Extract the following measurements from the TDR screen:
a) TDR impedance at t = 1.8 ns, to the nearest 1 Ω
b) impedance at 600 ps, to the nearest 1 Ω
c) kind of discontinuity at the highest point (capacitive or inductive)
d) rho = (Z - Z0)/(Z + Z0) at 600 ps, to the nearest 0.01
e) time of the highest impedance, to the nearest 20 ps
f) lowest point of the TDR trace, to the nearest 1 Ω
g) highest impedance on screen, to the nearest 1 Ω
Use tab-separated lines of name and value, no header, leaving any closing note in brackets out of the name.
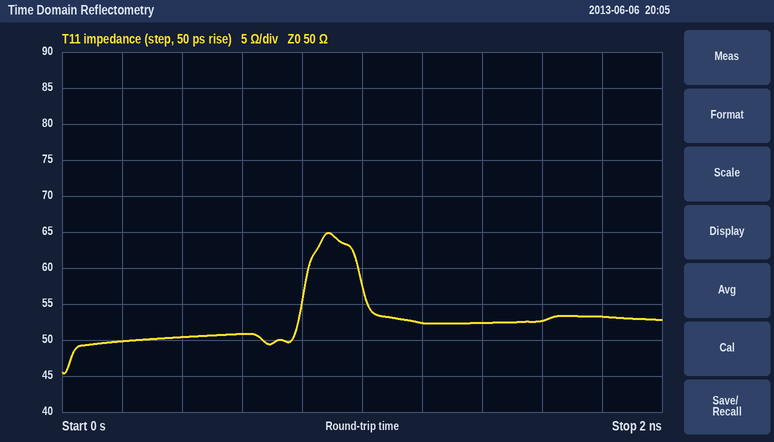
TDR impedance at t = 1.8 ns, to the nearest 1 Ω	53 Ω
impedance at 600 ps, to the nearest 1 Ω	51 Ω
kind of discontinuity at the highest point	inductive
rho = (Z - Z0)/(Z + Z0) at 600 ps, to the nearest 0.01	+0.01
time of the highest impedance, to the nearest 20 ps	880 ps
lowest point of the TDR trace, to the nearest 1 Ω	45 Ω
highest impedance on screen, to the nearest 1 Ω	65 Ω
